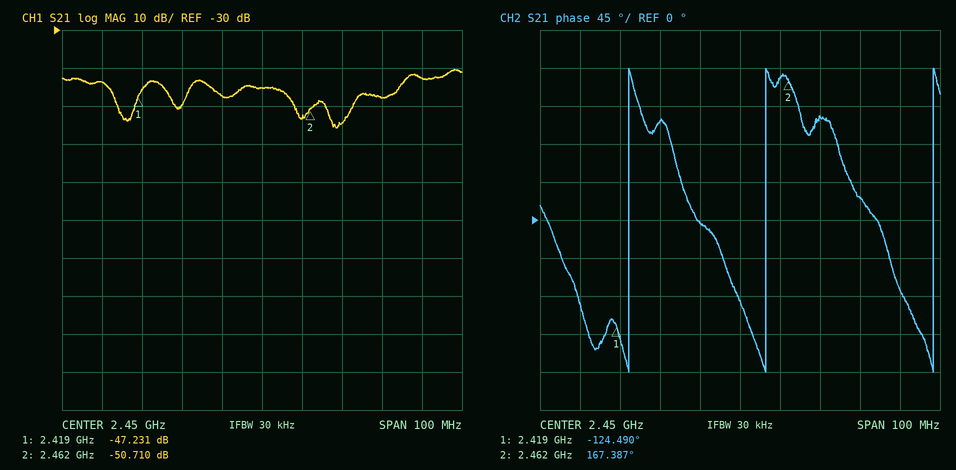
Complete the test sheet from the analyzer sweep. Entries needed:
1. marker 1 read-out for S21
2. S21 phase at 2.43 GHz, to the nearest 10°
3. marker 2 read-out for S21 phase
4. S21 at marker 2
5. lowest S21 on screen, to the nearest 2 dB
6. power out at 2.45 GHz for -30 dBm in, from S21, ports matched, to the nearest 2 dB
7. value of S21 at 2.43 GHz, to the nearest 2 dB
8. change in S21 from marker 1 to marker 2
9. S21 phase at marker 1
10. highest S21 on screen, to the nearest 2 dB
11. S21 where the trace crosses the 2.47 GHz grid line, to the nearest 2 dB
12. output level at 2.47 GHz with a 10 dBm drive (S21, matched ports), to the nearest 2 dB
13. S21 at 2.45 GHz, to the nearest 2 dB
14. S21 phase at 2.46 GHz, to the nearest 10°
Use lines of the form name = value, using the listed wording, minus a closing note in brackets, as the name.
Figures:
marker 1 read-out for S21 = -47.231 dB
S21 phase at 2.43 GHz, to the nearest 10° = 120°
marker 2 read-out for S21 phase = 167.387°
S21 at marker 2 = -50.710 dB
lowest S21 on screen, to the nearest 2 dB = -56 dB
power out at 2.45 GHz for -30 dBm in, from S21, ports matched, to the nearest 2 dB = -76 dBm
value of S21 at 2.43 GHz, to the nearest 2 dB = -50 dB
change in S21 from marker 1 to marker 2 = -3.479 dB
S21 phase at marker 1 = -124.490°
highest S21 on screen, to the nearest 2 dB = -40 dB
S21 where the trace crosses the 2.47 GHz grid line, to the nearest 2 dB = -54 dB
output level at 2.47 GHz with a 10 dBm drive (S21, matched ports), to the nearest 2 dB = -44 dBm
S21 at 2.45 GHz, to the nearest 2 dB = -46 dB
S21 phase at 2.46 GHz, to the nearest 10° = 170°
